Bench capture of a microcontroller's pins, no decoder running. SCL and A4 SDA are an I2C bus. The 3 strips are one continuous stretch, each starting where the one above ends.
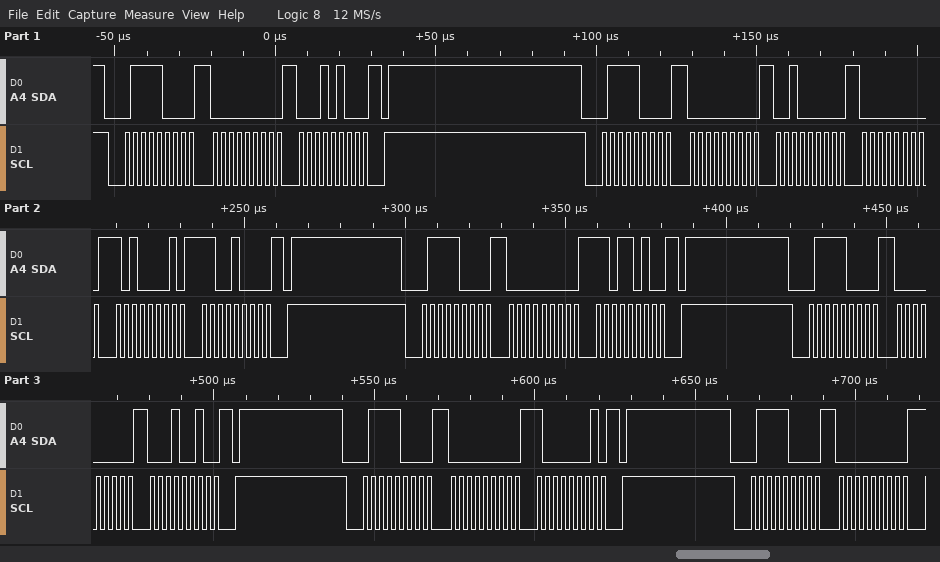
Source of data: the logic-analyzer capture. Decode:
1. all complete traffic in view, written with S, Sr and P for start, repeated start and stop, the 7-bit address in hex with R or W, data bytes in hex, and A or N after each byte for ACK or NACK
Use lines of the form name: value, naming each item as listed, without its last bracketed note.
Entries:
all complete traffic in view, written with S, Sr and P for start, repeated start and stop, the 7-bit address in hex with R or W, data bytes in hex, and A or N after each byte for ACK or NACK: S 3CW A 00 A 14 A P S 3CW A 00 A 20 A 00 A A1 A C8 A P S 3CW A 00 A DA A P S 3CW A 00 A 12 A P S 3CW A 00 A 81 A P S 3CW A 00 A
